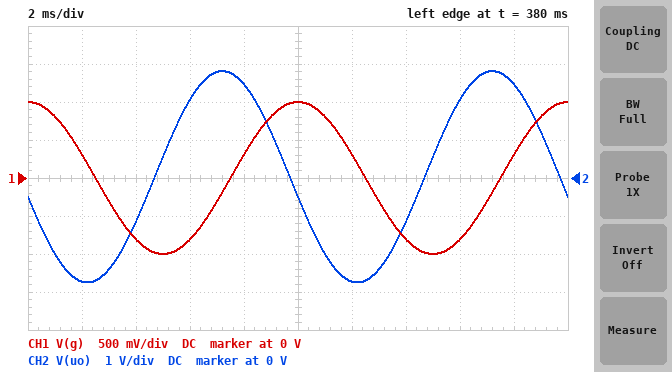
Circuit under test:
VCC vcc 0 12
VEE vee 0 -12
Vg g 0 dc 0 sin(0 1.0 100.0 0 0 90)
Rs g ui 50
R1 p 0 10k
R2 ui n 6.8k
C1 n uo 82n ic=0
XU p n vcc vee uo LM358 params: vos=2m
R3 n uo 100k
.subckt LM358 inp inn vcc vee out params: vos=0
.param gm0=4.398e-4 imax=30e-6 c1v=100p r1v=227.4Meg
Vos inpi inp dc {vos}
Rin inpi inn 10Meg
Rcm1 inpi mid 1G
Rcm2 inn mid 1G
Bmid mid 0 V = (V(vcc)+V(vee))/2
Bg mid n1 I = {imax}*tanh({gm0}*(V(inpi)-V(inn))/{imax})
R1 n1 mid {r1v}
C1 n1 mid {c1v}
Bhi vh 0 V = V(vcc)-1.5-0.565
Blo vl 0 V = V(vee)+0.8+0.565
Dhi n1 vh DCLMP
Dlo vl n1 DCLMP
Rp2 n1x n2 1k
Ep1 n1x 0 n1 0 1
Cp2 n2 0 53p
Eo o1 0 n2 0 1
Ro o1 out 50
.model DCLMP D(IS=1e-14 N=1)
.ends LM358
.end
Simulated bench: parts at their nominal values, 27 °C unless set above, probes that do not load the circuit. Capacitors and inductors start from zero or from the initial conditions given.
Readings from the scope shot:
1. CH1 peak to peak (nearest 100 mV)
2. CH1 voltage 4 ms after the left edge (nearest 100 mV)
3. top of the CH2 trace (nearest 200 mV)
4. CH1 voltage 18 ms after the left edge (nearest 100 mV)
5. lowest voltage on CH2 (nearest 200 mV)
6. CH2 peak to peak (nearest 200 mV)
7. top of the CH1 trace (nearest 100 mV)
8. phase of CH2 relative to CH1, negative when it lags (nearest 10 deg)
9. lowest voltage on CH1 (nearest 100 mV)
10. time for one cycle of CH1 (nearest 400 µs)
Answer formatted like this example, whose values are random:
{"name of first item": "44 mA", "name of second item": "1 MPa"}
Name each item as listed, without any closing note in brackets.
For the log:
{"CH1 peak to peak": "2.0 V", "CH1 voltage 4 ms after the left edge": "-800 mV", "top of the CH2 trace": "2.8 V", "CH1 voltage 18 ms after the left edge": "300 mV", "lowest voltage on CH2": "-2.8 V", "CH2 peak to peak": "5.6 V", "top of the CH1 trace": "1.0 V", "phase of CH2 relative to CH1, negative when it lags": "100 deg", "lowest voltage on CH1": "-1.0 V", "time for one cycle of CH1": "10.0 ms"}
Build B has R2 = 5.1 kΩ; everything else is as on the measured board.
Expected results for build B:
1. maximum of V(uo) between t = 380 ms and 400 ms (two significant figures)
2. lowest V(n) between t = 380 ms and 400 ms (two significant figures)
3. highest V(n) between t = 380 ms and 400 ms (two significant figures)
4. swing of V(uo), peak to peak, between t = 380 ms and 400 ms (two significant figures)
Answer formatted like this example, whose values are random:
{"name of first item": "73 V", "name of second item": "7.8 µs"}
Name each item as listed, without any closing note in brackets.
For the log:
{"maximum of V(uo) between t = 380 ms and 400 ms": "3.7 V", "lowest V(n) between t = 380 ms and 400 ms": "1.5 mV", "highest V(n) between t = 380 ms and 400 ms": "2.5 mV", "swing of V(uo), peak to peak, between t = 380 ms and 400 ms": "7.4 V"}
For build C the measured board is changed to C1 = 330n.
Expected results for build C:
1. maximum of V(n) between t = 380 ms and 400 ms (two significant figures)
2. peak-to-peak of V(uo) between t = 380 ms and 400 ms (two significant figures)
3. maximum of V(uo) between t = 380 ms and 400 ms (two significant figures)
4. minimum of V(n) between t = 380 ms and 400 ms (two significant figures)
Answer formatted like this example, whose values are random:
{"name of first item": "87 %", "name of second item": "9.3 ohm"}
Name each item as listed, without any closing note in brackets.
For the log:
{"maximum of V(n) between t = 380 ms and 400 ms": "2.1 mV", "peak-to-peak of V(uo) between t = 380 ms and 400 ms": "1.4 V", "maximum of V(uo) between t = 380 ms and 400 ms": "730 mV", "minimum of V(n) between t = 380 ms and 400 ms": "1.9 mV"}
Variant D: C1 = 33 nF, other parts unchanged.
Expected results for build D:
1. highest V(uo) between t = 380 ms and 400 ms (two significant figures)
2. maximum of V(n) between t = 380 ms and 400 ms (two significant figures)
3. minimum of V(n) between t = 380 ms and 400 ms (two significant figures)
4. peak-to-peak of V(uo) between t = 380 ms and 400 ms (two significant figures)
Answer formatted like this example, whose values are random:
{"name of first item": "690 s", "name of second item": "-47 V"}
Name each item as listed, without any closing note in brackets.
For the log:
{"highest V(uo) between t = 380 ms and 400 ms": "6.4 V", "maximum of V(n) between t = 380 ms and 400 ms": "2.9 mV", "minimum of V(n) between t = 380 ms and 400 ms": "1.1 mV", "peak-to-peak of V(uo) between t = 380 ms and 400 ms": "13 V"}
